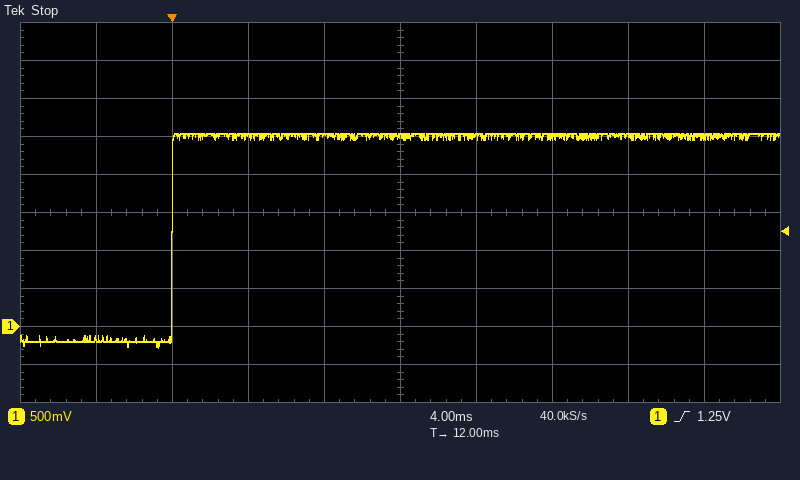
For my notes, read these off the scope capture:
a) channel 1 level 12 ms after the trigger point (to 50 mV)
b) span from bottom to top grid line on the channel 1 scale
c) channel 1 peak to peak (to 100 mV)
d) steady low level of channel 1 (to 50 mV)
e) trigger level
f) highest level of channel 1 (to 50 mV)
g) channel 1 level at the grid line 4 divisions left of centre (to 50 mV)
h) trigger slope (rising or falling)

2.50 V
5 V
2.80 V
-200 mV
1.25 V
2.55 V
-150 mV
rising
